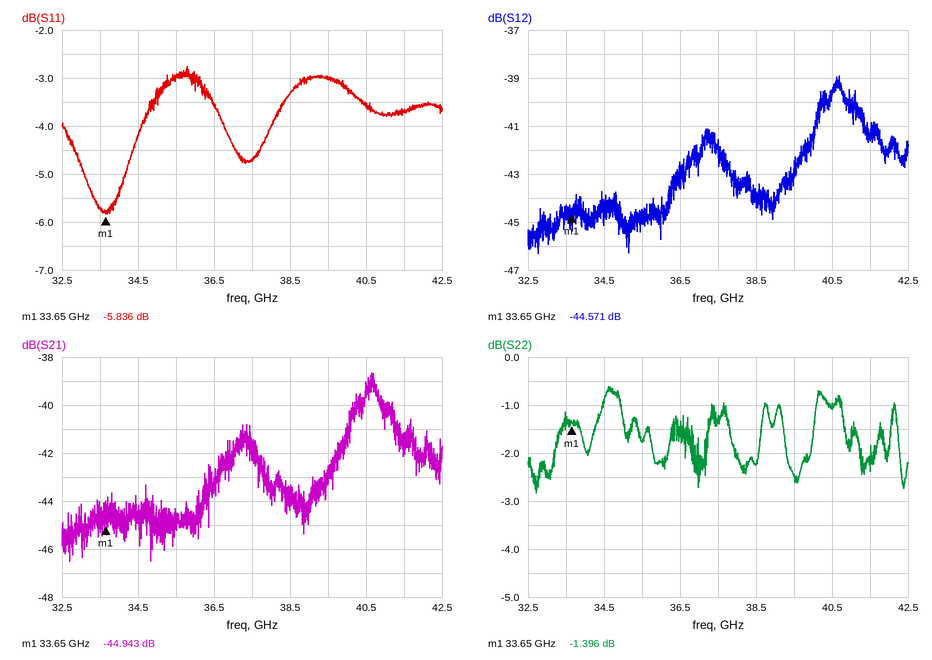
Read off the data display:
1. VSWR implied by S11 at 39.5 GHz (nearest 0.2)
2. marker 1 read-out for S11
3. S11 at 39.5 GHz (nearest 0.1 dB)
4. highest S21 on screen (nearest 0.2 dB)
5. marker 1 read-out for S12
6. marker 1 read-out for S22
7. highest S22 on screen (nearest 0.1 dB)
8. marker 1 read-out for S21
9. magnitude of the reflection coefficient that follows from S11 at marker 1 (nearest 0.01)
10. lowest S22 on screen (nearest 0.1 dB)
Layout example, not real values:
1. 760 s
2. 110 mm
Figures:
1. 5.8
2. -5.836 dB
3. -3.0 dB
4. -38.6 dB
5. -44.571 dB
6. -1.396 dB
7. -0.6 dB
8. -44.943 dB
9. 0.51
10. -2.8 dB
